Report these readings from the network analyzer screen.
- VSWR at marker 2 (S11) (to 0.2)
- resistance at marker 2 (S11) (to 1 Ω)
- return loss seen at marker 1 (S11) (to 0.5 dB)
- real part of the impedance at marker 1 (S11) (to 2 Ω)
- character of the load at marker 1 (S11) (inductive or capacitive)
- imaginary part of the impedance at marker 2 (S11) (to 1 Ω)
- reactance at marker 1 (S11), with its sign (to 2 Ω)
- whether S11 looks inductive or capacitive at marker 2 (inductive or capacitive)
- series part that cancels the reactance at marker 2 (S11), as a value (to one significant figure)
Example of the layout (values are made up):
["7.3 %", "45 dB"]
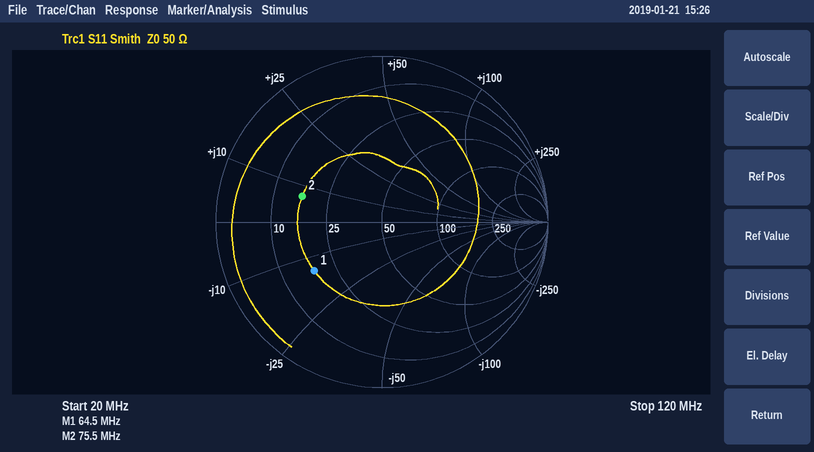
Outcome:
["3.0", "17 Ω", "6.0 dB", "18 Ω", "capacitive", "+7 Ω", "-14 Ω", "inductive", "300 pF"]
